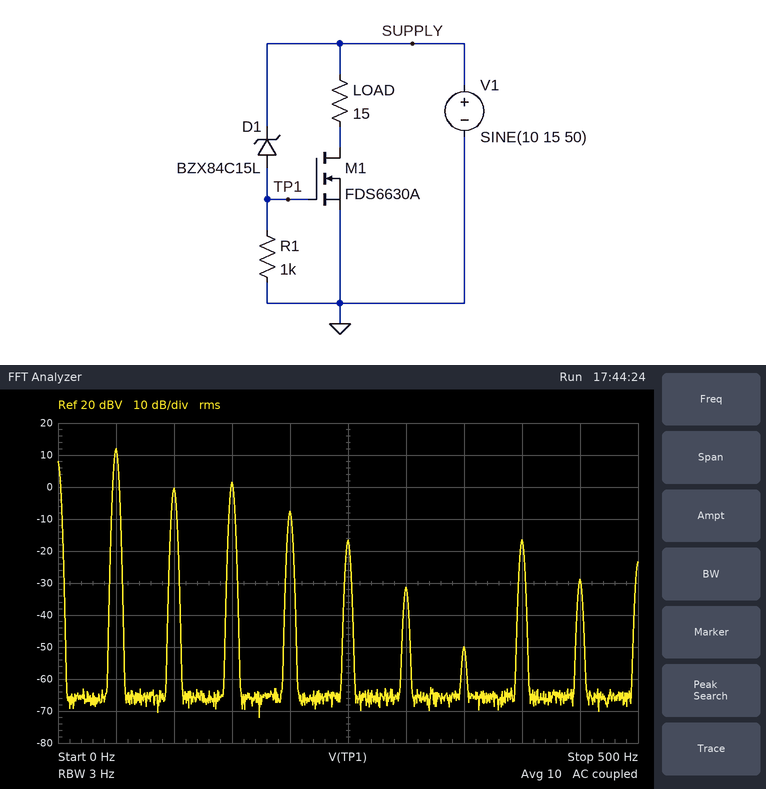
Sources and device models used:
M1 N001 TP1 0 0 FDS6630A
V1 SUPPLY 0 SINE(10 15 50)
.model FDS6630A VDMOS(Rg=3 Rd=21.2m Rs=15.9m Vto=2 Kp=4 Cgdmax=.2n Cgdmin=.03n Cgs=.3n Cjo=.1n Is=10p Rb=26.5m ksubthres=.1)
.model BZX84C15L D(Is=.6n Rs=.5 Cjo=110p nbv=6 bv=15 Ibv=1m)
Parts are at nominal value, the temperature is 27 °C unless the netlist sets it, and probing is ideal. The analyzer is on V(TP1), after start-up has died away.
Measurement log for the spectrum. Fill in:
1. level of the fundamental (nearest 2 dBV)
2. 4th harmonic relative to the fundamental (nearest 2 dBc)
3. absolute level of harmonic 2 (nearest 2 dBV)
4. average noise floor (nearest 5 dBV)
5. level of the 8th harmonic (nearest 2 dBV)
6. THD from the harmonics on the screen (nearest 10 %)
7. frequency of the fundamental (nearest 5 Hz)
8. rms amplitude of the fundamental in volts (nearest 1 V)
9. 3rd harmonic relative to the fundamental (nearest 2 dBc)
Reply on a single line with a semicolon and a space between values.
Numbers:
12 dBV; -20 dBc; 0 dBV; -65 dBV; -16 dBV; 40 %; 50 Hz; 4 V; -10 dBc
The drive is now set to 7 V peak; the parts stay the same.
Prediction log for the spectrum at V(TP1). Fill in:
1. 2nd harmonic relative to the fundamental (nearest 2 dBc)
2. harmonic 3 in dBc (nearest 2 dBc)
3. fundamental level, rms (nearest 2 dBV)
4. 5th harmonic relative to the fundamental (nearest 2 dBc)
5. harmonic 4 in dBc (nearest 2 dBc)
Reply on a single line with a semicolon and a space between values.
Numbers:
-2 dBc; -6 dBc; -8 dBV; -22 dBc; -10 dBc
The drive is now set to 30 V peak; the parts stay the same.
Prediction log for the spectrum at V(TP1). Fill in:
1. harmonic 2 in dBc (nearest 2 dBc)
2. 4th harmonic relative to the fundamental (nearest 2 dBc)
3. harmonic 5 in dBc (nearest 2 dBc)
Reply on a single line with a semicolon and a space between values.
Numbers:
-28 dBc; -30 dBc; -24 dBc
